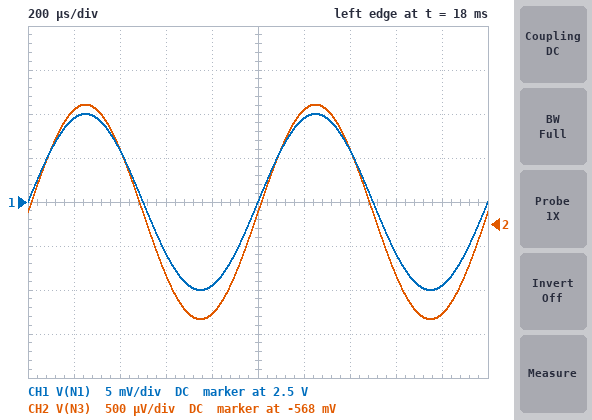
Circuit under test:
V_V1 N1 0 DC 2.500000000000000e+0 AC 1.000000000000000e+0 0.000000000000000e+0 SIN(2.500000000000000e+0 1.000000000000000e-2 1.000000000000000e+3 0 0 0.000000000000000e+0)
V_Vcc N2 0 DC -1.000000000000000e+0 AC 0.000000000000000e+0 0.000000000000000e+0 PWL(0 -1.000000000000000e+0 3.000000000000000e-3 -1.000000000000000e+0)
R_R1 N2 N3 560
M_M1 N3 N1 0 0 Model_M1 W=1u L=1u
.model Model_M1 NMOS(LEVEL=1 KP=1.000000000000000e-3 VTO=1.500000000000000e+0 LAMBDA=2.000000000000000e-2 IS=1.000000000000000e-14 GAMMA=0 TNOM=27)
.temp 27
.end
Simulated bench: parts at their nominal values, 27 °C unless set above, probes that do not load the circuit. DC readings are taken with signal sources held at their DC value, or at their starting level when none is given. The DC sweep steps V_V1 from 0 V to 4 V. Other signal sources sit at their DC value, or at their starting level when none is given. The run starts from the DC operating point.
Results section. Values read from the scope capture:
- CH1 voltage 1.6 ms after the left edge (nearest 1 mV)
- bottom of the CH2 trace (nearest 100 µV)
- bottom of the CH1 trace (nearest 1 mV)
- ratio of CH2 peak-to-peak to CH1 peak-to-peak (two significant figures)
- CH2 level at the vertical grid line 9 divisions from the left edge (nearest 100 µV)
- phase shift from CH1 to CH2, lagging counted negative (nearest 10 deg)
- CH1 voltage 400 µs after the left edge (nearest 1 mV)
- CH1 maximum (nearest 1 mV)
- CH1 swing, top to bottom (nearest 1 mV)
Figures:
2.494 V
-569.1 mV
2.490 V
0.12
-569.0 mV
0 deg
2.506 V
2.510 V
20 mV
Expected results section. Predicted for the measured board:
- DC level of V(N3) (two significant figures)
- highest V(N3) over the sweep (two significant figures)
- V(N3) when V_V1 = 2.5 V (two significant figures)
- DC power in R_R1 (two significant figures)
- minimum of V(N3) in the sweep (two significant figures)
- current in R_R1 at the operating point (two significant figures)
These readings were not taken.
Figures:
-570 mV
-400 mV
-570 mV
330 µW
-640 mV
770 µA
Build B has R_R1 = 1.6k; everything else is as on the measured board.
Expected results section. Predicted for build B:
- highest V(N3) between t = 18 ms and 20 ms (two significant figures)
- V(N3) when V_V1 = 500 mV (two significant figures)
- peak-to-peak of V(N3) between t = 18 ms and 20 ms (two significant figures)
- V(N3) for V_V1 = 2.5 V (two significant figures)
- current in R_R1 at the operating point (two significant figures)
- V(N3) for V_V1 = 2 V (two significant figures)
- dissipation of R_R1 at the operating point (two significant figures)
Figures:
-340 mV
-620 mV
3.5 mV
-350 mV
410 µA
-460 mV
270 µW
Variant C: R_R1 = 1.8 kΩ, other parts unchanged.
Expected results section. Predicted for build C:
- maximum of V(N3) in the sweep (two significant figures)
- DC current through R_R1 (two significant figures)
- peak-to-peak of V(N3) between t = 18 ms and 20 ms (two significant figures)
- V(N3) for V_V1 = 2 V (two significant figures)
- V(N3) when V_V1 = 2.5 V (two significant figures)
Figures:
-180 mV
380 µA
3.4 mV
-430 mV
-320 mV
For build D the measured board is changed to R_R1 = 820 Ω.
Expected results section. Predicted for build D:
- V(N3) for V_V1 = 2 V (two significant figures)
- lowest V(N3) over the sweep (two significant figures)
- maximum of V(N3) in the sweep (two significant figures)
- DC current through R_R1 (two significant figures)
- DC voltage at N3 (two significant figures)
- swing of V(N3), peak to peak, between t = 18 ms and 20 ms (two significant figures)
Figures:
-580 mV
-630 mV
-310 mV
620 µA
-490 mV
3.5 mV
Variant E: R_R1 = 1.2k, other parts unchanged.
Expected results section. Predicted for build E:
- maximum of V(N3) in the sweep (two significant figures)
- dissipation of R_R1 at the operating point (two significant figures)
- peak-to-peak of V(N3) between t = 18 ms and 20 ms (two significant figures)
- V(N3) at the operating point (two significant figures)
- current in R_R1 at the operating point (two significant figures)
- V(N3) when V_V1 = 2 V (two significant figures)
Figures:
-240 mV
290 µW
3.6 mV
-410 mV
490 µA
-520 mV
